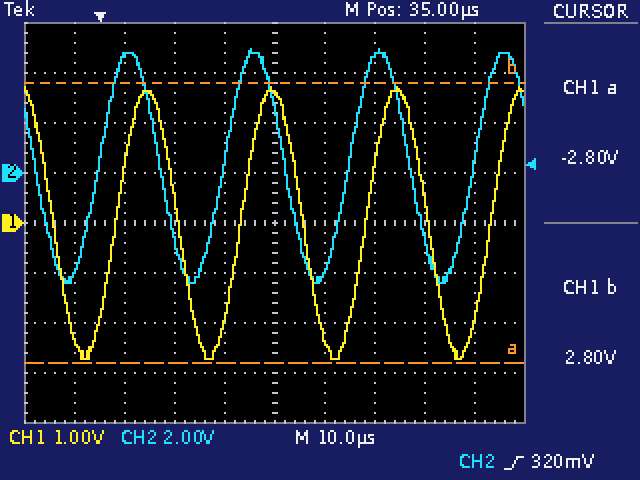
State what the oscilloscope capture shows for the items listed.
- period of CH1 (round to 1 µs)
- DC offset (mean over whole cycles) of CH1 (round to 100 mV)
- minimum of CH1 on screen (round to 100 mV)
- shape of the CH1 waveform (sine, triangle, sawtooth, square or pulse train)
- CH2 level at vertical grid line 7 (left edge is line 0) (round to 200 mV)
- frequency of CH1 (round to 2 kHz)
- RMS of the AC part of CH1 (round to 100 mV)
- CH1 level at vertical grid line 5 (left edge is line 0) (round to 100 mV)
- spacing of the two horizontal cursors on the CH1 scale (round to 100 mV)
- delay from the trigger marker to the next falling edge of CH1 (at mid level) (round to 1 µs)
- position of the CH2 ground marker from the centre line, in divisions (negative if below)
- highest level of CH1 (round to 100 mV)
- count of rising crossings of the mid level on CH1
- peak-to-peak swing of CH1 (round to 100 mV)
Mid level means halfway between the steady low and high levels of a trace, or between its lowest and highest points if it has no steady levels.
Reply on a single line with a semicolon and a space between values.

25 µs; 0.0 V; -2.7 V; sine; 4.6 V; 40 kHz; 1.9 V; 2.6 V; 5.6 V; 16 µs; +1.0 div; 2.7 V; 4; 5.4 V
